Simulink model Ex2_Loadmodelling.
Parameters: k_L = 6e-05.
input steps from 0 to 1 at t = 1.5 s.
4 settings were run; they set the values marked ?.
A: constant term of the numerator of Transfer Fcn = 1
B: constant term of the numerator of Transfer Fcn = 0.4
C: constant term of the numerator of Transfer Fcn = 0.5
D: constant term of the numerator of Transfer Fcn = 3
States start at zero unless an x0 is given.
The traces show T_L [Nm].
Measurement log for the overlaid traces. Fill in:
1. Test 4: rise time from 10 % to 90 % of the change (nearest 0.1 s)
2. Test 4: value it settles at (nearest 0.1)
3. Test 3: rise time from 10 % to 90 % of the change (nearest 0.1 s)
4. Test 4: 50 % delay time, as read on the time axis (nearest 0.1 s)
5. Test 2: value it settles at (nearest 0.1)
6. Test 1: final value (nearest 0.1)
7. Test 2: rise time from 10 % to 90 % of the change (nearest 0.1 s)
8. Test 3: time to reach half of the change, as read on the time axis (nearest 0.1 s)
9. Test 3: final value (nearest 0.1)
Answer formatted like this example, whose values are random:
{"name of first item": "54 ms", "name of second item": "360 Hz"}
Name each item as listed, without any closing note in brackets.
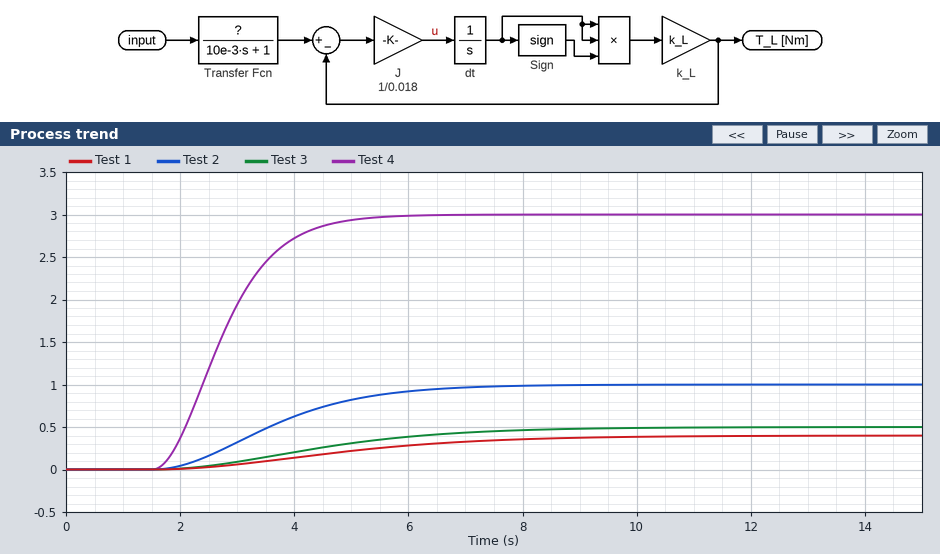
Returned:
{"Test 4: rise time from 10 % to 90 % of the change": "2.0 s", "Test 4: value it settles at": "3.0", "Test 3: rise time from 10 % to 90 % of the change": "4.9 s", "Test 4: 50 % delay time, as read on the time axis": "2.7 s", "Test 2: value it settles at": "1.0", "Test 1: final value": "0.4", "Test 2: rise time from 10 % to 90 % of the change": "3.5 s", "Test 3: time to reach half of the change, as read on the time axis": "4.4 s", "Test 3: final value": "0.5"}
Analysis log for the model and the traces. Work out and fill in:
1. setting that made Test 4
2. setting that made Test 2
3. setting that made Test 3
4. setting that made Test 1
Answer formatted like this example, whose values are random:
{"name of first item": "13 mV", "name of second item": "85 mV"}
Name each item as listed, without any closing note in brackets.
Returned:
{"setting that made Test 4": "D", "setting that made Test 2": "A", "setting that made Test 3": "C", "setting that made Test 1": "B"}
